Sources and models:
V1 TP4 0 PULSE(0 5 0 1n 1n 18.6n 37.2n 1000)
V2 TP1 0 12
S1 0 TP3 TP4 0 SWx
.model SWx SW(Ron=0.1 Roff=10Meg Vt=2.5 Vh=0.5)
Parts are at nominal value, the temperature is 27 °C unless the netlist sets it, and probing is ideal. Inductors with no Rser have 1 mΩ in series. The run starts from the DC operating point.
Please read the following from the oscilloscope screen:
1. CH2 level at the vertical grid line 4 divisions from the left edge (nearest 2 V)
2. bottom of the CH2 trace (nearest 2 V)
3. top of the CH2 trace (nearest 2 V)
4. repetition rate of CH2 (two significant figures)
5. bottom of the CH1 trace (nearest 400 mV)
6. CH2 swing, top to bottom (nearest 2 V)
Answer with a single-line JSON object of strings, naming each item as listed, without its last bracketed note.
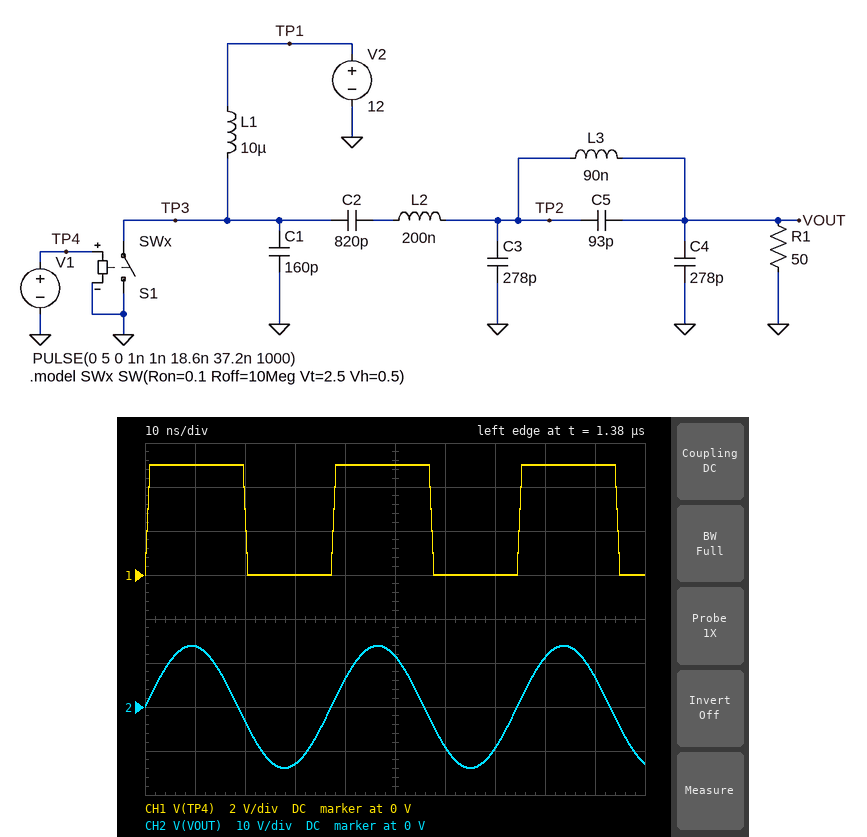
{"CH2 level at the vertical grid line 4 divisions from the left edge": "6 V", "bottom of the CH2 trace": "-14 V", "top of the CH2 trace": "14 V", "repetition rate of CH2": "27 MHz", "bottom of the CH1 trace": "0 V", "CH2 swing, top to bottom": "28 V"}
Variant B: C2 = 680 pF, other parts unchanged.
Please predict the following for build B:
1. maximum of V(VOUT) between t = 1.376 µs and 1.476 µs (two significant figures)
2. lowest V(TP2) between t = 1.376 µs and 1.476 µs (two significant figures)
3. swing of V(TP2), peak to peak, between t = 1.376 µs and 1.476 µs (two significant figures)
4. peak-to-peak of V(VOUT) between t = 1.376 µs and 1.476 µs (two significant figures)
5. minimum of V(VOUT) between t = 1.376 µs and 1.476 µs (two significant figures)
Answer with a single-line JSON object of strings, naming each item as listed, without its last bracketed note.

{"maximum of V(VOUT) between t = 1.376 µs and 1.476 µs": "15 V", "lowest V(TP2) between t = 1.376 µs and 1.476 µs": "-5.0 V", "swing of V(TP2), peak to peak, between t = 1.376 µs and 1.476 µs": "13 V", "peak-to-peak of V(VOUT) between t = 1.376 µs and 1.476 µs": "29 V", "minimum of V(VOUT) between t = 1.376 µs and 1.476 µs": "-15 V"}
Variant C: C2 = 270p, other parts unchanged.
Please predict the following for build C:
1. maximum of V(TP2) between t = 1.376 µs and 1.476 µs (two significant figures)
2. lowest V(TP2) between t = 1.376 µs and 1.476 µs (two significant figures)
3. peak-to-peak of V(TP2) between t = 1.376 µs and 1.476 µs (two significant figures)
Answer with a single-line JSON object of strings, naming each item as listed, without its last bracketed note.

{"maximum of V(TP2) between t = 1.376 µs and 1.476 µs": "13 V", "lowest V(TP2) between t = 1.376 µs and 1.476 µs": "-11 V", "peak-to-peak of V(TP2) between t = 1.376 µs and 1.476 µs": "23 V"}
